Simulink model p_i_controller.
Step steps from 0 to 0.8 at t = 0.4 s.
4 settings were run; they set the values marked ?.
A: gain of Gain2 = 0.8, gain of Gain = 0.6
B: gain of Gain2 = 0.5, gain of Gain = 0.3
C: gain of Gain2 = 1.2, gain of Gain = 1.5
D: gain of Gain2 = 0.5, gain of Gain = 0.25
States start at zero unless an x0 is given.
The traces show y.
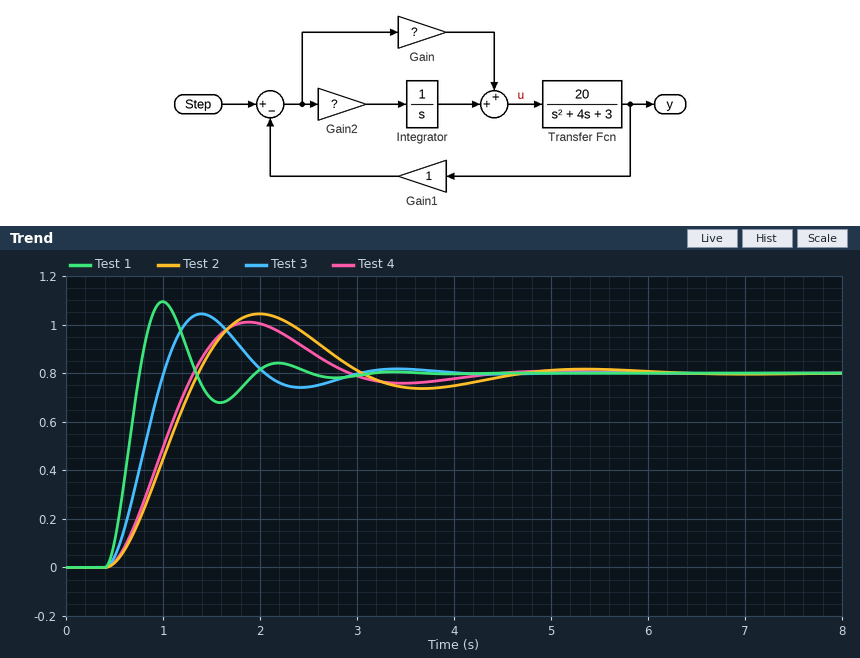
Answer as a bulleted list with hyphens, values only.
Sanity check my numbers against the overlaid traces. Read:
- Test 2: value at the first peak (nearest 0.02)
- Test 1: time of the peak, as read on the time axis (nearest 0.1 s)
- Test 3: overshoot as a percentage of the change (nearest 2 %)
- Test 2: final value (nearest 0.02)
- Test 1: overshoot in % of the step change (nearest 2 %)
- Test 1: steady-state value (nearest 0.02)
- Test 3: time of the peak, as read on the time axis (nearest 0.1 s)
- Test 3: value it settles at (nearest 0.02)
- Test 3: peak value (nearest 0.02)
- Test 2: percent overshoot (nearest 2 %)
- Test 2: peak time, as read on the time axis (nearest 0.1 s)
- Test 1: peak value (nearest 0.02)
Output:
- 1.04
- 1.0 s
- 30 %
- 0.80
- 36 %
- 0.80
- 1.4 s
- 0.80
- 1.04
- 30 %
- 2.0 s
- 1.10
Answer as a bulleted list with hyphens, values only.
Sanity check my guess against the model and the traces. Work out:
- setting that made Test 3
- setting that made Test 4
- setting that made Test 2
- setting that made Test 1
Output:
- A
- B
- D
- C
